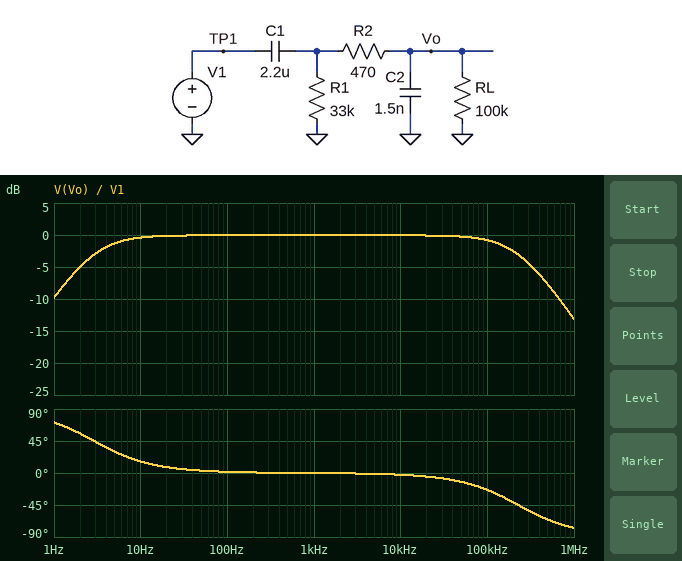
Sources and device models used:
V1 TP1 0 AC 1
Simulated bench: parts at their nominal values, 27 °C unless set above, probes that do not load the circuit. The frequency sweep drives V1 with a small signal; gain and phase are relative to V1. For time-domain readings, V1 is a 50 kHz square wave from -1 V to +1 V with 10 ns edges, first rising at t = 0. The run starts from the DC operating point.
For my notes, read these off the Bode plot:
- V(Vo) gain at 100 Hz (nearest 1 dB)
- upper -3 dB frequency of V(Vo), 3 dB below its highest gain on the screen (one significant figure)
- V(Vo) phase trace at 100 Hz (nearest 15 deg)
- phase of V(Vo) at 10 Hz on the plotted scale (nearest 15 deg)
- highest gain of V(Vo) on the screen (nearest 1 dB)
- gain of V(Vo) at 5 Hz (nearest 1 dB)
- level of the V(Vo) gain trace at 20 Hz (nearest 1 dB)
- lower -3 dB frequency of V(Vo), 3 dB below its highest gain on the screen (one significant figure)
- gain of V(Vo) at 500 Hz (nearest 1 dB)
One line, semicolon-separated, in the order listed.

0 dB; 200 kHz; 0 deg; 15 deg; 0 dB; -1 dB; 0 dB; 3 Hz; 0 dB
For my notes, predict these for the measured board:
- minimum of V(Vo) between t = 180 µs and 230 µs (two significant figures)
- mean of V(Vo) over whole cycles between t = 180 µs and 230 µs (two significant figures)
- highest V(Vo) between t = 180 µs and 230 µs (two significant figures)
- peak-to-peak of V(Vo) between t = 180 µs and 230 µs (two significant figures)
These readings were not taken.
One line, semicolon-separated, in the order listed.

-4.0 mV; 990 mV; 2.0 V; 2.0 V
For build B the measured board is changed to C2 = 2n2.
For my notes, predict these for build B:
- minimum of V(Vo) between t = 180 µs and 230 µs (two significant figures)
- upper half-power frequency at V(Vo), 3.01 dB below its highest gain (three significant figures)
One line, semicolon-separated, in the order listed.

-3.9 mV; 155 kHz
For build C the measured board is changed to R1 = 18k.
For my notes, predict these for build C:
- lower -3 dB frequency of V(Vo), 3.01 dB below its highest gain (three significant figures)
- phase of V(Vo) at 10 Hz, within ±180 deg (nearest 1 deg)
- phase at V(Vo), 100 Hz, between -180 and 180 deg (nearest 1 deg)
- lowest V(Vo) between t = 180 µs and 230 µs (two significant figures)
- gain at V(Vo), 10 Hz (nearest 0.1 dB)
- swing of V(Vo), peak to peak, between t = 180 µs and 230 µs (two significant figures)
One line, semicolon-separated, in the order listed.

4.74 Hz; 25 deg; 3 deg; -6.5 mV; -0.9 dB; 2.0 V
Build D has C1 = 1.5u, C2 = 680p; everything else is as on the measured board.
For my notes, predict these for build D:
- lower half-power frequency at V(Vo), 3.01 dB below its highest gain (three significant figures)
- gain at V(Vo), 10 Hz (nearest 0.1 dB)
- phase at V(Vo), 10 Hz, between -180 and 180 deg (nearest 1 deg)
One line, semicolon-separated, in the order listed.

4.27 Hz; -0.8 dB; 23 deg
